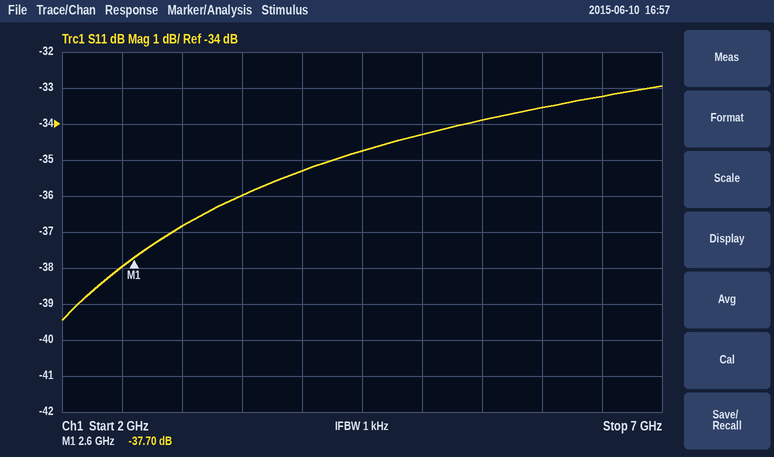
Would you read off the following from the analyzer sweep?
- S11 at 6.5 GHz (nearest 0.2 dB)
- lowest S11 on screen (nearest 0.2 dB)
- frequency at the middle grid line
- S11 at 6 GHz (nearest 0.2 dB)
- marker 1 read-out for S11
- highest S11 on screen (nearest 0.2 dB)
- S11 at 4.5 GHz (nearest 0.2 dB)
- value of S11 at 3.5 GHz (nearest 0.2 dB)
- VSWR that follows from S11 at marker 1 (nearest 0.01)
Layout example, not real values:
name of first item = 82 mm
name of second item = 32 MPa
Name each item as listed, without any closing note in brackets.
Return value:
S11 at 6.5 GHz = -33.2 dB
lowest S11 on screen = -39.4 dB
frequency at the middle grid line = 4.5 GHz
S11 at 6 GHz = -33.6 dB
marker 1 read-out for S11 = -37.70 dB
highest S11 on screen = -33.0 dB
S11 at 4.5 GHz = -34.8 dB
value of S11 at 3.5 GHz = -36.0 dB
VSWR that follows from S11 at marker 1 = 1.03
